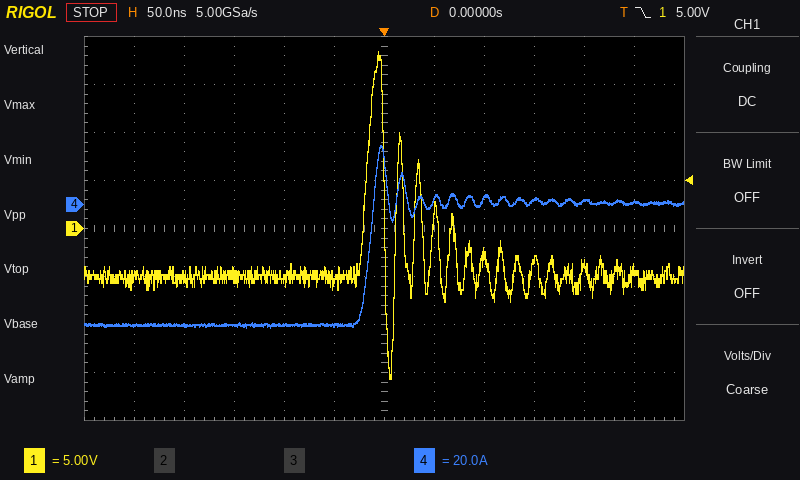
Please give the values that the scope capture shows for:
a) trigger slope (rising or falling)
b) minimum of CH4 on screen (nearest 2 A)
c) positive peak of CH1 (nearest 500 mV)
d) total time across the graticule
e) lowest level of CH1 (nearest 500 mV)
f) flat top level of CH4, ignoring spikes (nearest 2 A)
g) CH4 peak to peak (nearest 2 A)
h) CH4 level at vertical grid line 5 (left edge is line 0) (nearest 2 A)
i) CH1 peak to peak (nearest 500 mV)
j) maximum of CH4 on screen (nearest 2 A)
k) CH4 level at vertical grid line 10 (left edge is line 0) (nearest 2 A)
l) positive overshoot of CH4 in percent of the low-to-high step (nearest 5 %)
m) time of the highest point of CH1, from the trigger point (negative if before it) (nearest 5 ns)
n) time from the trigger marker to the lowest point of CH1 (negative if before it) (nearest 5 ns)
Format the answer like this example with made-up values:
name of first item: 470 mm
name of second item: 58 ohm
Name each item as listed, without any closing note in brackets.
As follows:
trigger slope: falling
minimum of CH4 on screen: -52 A
positive peak of CH1: 18.5 V
total time across the graticule: 600 ns
lowest level of CH1: -15.5 V
flat top level of CH4, ignoring spikes: 0 A
CH4 peak to peak: 76 A
CH4 level at vertical grid line 5 (left edge is line 0): -50 A
CH1 peak to peak: 34.0 V
maximum of CH4 on screen: 24 A
CH4 level at vertical grid line 10 (left edge is line 0): 2 A
positive overshoot of CH4 in percent of the low-to-high step: 45 %
time of the highest point of CH1, from the trigger point (negative if before it): -5 ns
time from the trigger marker to the lowest point of CH1 (negative if before it): +5 ns
